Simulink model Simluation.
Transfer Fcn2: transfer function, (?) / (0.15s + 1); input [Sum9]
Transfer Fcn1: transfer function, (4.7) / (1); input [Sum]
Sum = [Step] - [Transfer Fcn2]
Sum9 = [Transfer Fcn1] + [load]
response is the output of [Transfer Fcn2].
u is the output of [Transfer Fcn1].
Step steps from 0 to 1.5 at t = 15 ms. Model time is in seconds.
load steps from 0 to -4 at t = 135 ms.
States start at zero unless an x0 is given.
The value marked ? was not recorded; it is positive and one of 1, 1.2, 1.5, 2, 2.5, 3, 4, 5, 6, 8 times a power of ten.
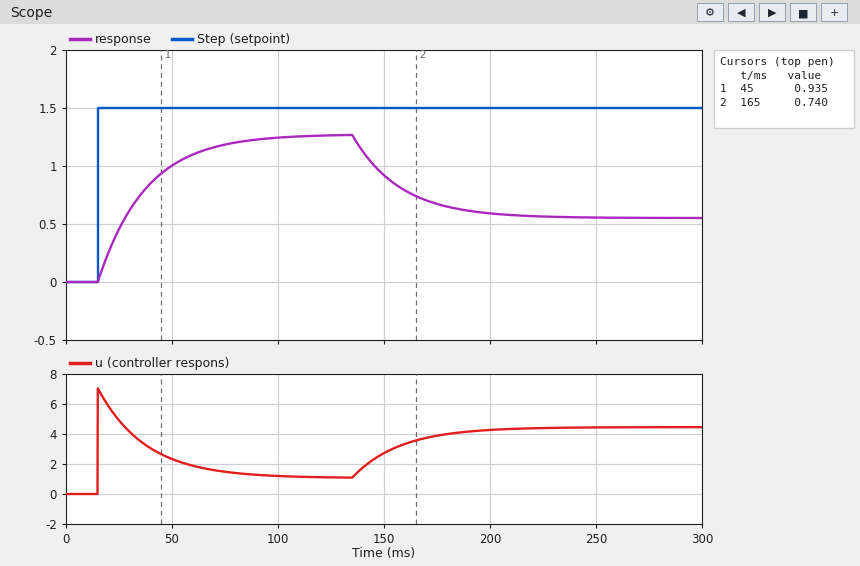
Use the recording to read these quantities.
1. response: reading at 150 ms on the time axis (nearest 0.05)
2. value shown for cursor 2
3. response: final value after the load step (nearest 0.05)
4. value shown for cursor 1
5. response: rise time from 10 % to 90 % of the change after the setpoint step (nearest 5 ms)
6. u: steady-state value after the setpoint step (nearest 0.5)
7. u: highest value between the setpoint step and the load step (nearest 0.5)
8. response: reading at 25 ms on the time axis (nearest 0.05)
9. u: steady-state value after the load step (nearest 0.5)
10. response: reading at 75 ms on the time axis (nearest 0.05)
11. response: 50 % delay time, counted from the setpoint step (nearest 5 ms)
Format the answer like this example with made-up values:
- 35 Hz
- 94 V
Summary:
- 0.90
- 0.740
- 0.55
- 0.935
- 50 ms
- 1.0
- 7.0
- 0.45
- 4.5
- 1.20
- 15 ms
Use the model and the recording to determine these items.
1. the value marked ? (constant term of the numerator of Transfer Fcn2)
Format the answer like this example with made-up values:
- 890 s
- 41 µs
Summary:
- 1.2
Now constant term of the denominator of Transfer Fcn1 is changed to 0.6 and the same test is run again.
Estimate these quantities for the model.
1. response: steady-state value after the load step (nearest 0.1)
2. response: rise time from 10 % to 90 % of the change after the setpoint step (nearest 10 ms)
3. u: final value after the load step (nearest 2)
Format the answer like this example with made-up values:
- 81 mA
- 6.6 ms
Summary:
- 0.9
- 30 ms
- 4
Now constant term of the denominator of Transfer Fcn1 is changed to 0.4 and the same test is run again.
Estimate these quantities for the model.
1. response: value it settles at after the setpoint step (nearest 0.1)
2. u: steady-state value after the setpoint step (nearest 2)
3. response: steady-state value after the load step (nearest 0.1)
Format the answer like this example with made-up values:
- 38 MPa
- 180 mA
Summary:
- 1.4
- 2
- 1.1
